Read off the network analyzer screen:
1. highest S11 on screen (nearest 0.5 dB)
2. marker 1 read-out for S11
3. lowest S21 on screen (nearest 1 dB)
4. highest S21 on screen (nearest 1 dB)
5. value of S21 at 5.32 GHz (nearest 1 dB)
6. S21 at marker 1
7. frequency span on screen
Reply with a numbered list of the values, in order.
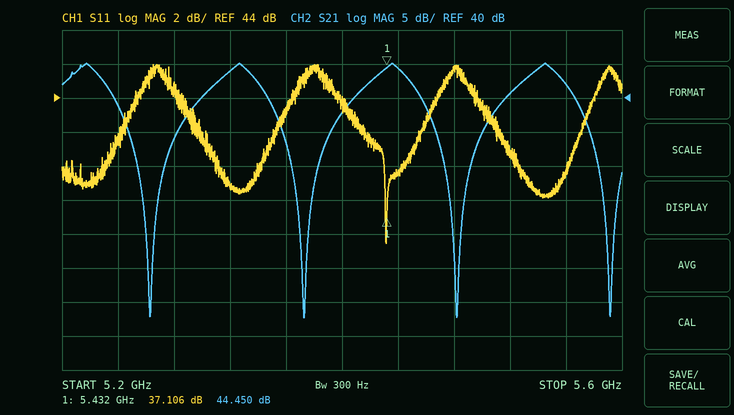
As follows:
1. 46.0 dB
2. 37.106 dB
3. 8 dB
4. 45 dB
5. 44 dB
6. 44.450 dB
7. 400 MHz
